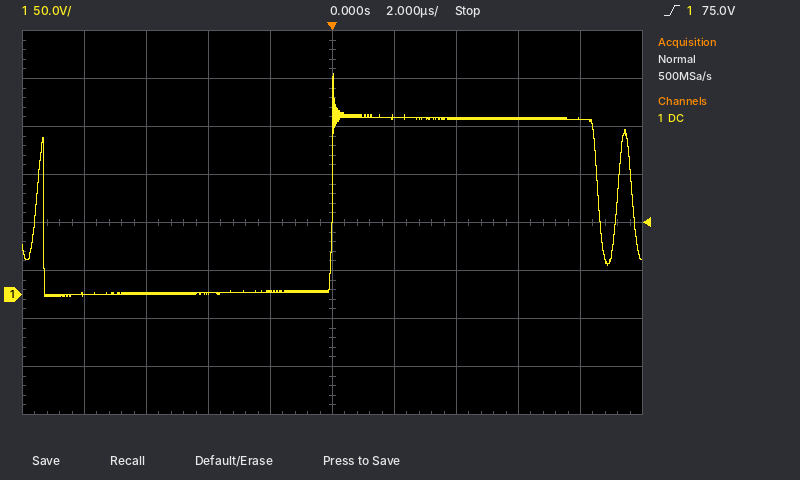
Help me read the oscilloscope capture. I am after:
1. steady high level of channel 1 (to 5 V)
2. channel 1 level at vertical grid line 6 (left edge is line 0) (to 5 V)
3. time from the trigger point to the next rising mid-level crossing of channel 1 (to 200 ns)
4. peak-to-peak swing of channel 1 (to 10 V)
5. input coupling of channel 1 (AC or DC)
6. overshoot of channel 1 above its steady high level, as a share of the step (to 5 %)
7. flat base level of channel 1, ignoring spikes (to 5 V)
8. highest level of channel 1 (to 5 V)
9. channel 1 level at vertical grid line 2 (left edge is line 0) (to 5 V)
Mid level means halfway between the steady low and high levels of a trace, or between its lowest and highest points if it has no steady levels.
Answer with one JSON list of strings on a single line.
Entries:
["185 V", "185 V", "9.2 µs", "230 V", "DC", "25 %", "0 V", "230 V", "0 V"]
